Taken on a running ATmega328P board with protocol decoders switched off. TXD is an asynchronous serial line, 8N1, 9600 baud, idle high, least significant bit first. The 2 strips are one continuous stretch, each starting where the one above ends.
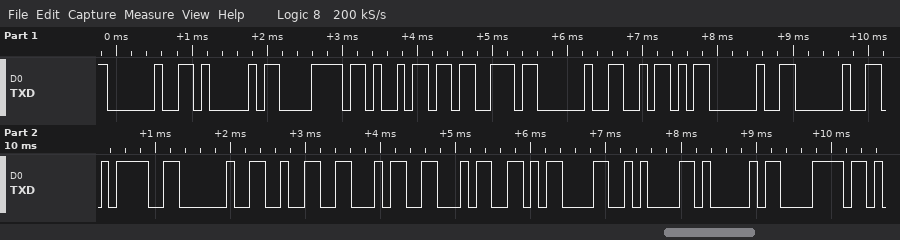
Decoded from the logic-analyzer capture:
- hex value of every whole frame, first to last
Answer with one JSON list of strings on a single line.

["20 41 78 69 73 20 5A 20 20 3D 20 32 34 34 0D 0A 41 78"]
